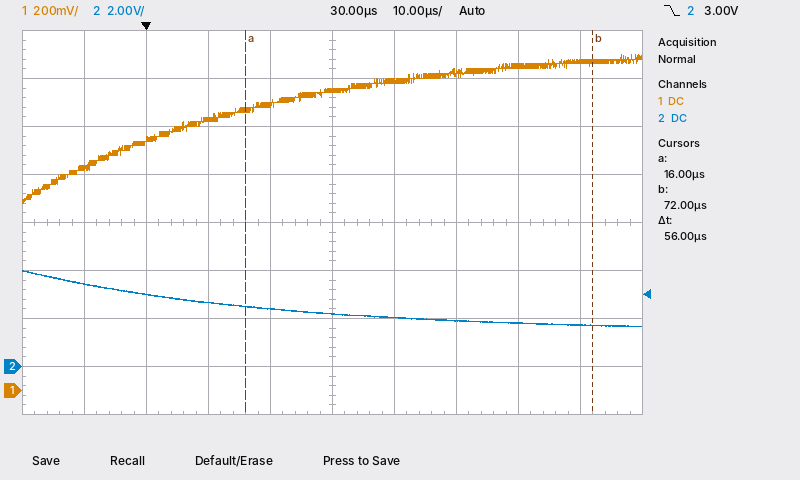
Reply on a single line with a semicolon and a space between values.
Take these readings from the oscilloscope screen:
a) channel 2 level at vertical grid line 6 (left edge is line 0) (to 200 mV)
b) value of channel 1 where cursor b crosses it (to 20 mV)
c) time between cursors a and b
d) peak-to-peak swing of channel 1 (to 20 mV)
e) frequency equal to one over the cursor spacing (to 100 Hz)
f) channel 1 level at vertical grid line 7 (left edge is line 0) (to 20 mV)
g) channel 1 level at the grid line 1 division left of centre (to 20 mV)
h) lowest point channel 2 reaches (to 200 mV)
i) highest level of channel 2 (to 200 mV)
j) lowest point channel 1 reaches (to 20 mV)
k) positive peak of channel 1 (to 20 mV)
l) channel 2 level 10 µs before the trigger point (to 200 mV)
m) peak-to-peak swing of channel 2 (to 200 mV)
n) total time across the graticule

2.0 V; 1.36 V; 56 µs; 620 mV; 17.9 kHz; 1.32 V; 1.20 V; 1.6 V; 4.0 V; 780 mV; 1.40 V; 3.4 V; 2.4 V; 100 µs
